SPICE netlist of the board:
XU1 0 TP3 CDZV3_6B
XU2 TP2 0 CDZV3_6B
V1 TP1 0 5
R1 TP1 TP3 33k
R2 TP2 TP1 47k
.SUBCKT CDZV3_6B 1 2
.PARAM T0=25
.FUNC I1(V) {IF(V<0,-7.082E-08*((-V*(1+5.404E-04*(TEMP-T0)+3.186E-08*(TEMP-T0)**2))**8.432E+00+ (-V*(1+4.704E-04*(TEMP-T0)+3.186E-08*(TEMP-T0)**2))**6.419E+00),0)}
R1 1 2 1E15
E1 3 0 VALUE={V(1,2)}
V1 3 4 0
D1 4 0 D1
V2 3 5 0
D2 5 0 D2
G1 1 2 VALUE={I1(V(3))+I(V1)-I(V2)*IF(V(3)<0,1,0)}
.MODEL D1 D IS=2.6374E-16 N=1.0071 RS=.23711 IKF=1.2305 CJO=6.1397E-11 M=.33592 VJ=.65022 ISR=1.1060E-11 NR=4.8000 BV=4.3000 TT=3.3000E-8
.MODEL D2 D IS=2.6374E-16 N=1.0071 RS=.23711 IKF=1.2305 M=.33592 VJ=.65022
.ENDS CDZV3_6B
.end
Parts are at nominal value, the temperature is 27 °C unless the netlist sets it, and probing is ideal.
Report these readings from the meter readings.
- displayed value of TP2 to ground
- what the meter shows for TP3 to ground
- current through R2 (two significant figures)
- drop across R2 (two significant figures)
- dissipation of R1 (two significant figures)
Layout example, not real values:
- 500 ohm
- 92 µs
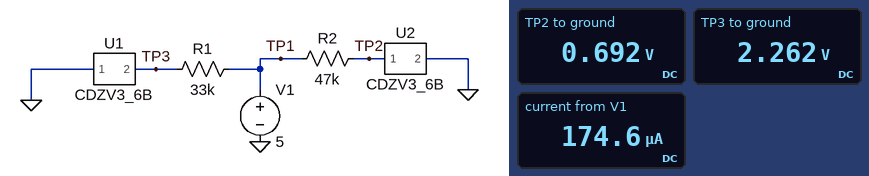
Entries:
- 0.692 V
- 2.262 V
- 92 µA
- 4.3 V
- 230 µW
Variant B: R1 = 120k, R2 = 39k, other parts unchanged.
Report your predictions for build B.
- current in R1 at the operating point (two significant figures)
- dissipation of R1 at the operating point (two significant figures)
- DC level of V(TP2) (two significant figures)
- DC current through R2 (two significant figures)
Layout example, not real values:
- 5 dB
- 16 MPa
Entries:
- 25 µA
- 77 µW
- 700 mV
- 110 µA
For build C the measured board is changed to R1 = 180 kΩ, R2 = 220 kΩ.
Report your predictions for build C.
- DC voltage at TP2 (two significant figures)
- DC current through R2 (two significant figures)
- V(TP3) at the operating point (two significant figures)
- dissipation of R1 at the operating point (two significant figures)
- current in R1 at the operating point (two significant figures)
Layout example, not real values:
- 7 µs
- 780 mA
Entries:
- 650 mV
- 20 µA
- 1.9 V
- 55 µW
- 17 µA
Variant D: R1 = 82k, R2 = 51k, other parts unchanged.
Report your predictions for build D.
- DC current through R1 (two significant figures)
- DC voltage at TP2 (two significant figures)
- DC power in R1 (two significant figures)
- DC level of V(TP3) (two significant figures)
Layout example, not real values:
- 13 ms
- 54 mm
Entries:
- 36 µA
- 690 mV
- 110 µW
- 2.0 V
